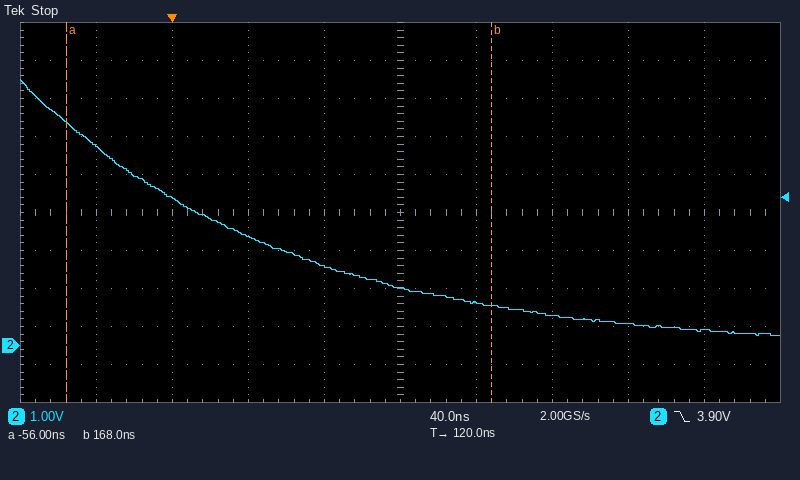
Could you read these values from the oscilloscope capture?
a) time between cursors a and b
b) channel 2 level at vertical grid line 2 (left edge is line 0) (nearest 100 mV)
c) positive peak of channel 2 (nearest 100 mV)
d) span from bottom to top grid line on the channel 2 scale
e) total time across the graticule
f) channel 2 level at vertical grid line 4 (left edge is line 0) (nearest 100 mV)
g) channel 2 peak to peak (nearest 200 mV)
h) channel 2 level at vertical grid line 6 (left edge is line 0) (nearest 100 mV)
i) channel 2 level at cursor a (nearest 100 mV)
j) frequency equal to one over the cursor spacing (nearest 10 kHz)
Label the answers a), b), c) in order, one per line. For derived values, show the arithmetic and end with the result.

a) 168 ns − (-56 ns) = 224 ns
b) 3.9 V
c) 7.0 V
d) 10 V
e) 400 ns
f) 2.1 V
g) 6.8 V
h) 1.1 V
i) 5.9 V
j) 1 / 224 ns ≈ 4.46 MHz
